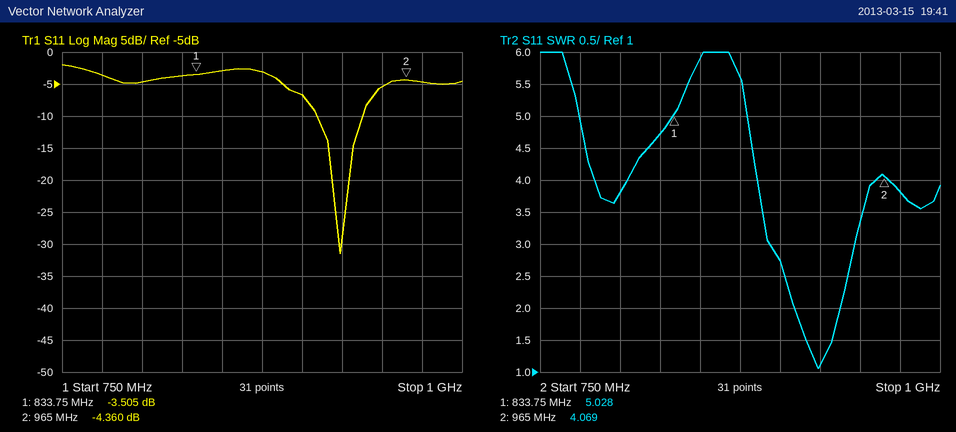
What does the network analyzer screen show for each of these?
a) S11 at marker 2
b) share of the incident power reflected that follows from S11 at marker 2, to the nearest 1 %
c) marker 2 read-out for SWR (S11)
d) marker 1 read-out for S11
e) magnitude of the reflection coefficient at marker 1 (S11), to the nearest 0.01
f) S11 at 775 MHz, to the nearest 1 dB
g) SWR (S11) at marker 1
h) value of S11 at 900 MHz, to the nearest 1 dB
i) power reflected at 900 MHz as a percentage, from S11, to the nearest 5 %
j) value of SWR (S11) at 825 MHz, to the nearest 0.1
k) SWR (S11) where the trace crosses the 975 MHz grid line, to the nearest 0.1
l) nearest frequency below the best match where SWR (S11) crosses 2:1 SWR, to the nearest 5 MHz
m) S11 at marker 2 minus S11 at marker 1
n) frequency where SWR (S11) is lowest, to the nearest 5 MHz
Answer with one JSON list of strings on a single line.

["-4.360 dB", "37 %", "4.069", "-3.505 dB", "0.67", "-4 dB", "5.028", "-7 dB", "20 %", "4.7", "3.8", "910 MHz", "-0.855 dB", "925 MHz"]
